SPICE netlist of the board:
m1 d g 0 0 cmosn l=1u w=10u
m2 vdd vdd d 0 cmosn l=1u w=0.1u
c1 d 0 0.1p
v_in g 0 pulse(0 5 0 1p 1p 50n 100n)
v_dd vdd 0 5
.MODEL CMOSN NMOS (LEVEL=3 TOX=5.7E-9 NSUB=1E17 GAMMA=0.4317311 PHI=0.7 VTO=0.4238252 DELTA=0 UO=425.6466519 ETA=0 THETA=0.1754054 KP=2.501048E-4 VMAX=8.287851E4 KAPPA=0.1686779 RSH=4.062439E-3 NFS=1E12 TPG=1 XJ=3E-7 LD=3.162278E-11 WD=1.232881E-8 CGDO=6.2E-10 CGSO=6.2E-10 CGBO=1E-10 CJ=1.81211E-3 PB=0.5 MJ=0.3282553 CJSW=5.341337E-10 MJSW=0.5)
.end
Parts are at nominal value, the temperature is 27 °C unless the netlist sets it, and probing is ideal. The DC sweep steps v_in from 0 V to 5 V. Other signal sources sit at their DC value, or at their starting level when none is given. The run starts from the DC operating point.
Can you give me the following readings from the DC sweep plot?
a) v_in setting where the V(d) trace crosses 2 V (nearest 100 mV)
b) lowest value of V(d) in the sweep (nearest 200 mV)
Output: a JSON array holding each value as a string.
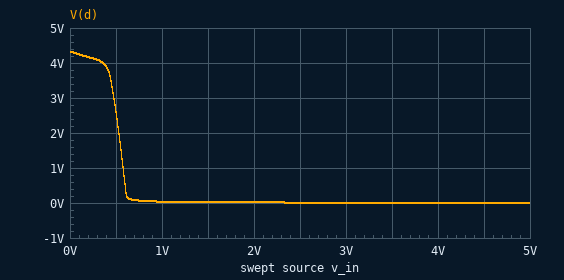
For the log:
["500 mV", "0 V"]
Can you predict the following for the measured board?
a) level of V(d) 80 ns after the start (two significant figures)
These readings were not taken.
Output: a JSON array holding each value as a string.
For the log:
["3.6 V"]
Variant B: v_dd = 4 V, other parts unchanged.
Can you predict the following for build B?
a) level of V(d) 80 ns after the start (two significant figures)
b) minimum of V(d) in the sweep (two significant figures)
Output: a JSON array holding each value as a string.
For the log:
["2.7 V", "5.8 mV"]
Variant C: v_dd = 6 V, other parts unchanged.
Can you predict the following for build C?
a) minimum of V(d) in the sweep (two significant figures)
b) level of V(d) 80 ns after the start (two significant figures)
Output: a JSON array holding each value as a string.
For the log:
["10 mV", "4.5 V"]
